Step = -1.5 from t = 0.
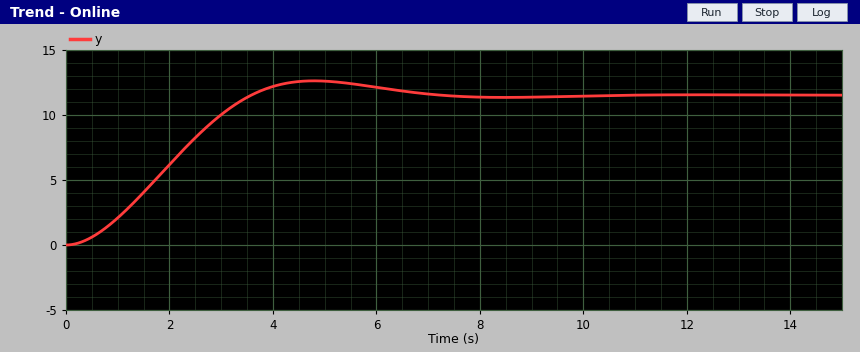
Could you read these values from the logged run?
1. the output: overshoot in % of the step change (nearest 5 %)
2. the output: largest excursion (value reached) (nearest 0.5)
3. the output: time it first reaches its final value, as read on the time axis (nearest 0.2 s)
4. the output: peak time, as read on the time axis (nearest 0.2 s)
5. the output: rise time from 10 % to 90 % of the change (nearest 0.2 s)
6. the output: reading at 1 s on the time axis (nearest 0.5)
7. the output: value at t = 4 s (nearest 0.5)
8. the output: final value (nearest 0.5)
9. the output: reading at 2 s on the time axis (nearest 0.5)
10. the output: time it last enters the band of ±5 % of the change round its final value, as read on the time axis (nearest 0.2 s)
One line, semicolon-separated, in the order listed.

10 %; 12.5; 3.6 s; 4.8 s; 2.4 s; 2.0; 12.0; 11.5; 6.0; 6.0 s
